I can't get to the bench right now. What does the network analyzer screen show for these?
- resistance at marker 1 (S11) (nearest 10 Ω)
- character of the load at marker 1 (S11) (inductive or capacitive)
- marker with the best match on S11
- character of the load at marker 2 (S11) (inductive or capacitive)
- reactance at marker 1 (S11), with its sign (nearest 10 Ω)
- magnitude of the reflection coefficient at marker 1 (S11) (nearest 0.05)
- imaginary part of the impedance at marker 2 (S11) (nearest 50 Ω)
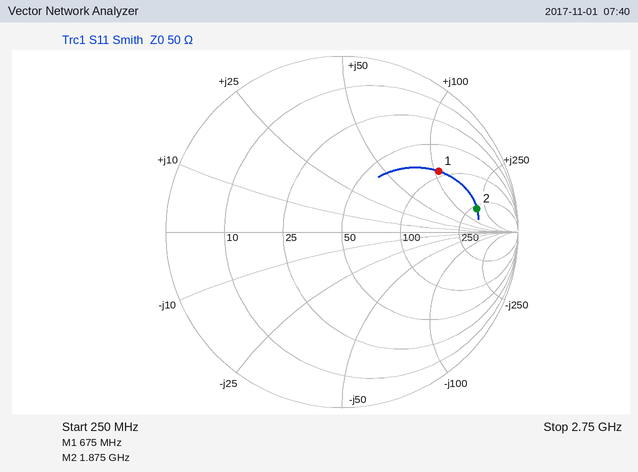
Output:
90 Ω
inductive
marker 1
inductive
+110 Ω
0.65
+200 Ω
